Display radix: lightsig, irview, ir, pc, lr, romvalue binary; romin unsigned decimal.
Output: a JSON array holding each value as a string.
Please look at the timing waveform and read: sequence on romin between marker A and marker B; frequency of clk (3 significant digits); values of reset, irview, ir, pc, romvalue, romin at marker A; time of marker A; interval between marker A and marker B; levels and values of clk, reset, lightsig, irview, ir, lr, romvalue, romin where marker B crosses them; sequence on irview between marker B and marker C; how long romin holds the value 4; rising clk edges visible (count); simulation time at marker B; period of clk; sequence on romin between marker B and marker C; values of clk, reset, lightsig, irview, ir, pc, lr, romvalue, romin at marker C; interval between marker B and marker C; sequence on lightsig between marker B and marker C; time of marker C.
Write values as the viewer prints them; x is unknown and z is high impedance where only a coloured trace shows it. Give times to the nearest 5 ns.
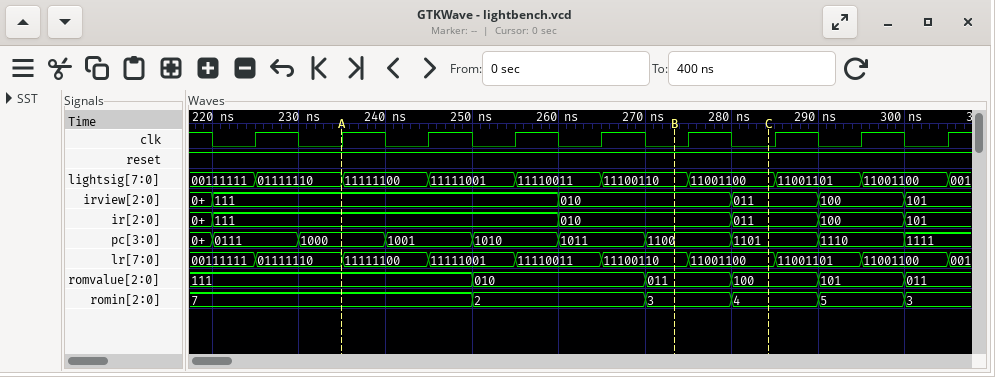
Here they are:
["7, 2, 3", "100 MHz", "reset=1, irview=111, ir=111, pc=1000, romvalue=111, romin=7", "235 ns", "40 ns", "clk=0, reset=1, lightsig=11100110, irview=010, ir=010, lr=11100110, romvalue=011, romin=3", "010, 011", "10 ns", "9", "275 ns", "10 ns", "3, 4", "clk=0, reset=1, lightsig=11001100, irview=011, ir=011, pc=1101, lr=11001100, romvalue=100, romin=4", "10 ns", "11100110, 11001100", "285 ns"]
